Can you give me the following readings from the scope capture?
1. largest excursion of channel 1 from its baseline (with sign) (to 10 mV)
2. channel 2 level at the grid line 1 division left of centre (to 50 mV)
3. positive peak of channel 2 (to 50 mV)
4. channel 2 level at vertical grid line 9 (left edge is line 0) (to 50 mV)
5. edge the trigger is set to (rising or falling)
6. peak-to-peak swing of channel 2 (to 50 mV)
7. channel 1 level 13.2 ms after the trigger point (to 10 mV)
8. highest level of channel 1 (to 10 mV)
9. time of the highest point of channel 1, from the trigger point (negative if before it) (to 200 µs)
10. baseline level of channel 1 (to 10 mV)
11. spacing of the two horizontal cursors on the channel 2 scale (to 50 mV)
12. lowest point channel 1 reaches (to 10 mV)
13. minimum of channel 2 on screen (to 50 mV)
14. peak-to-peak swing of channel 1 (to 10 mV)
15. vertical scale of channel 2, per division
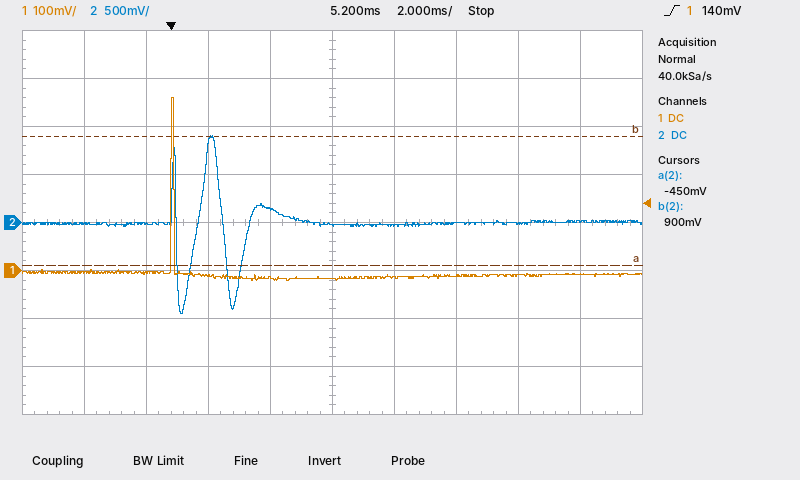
+370 mV
150 mV
900 mV
0 mV
rising
1.85 V
-10 mV
360 mV
0.0 ms
-10 mV
1.35 V
-20 mV
-950 mV
380 mV
500 mV
